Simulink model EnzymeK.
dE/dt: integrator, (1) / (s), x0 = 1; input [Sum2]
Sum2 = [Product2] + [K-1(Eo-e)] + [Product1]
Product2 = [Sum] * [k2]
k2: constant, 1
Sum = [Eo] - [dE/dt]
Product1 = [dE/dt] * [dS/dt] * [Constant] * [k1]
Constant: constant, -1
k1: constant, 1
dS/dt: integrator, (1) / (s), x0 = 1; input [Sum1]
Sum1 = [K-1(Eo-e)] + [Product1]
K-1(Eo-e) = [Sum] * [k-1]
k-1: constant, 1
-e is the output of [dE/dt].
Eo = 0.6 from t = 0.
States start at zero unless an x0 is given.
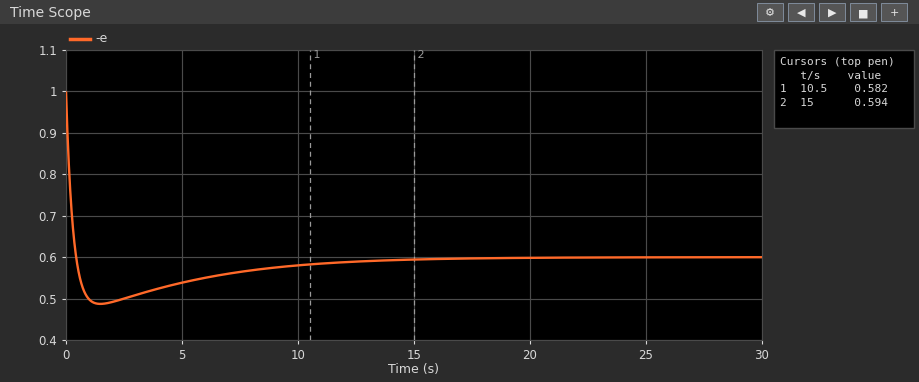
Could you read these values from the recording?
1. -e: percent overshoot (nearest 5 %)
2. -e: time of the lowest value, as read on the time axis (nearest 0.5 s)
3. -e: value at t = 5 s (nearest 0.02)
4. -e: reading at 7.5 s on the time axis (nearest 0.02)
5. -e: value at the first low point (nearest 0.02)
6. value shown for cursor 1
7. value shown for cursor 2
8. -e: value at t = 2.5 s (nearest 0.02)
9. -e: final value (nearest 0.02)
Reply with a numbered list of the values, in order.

1. 30 %
2. 1.5 s
3. 0.54
4. 0.56
5. 0.48
6. 0.582
7. 0.594
8. 0.50
9. 0.60
